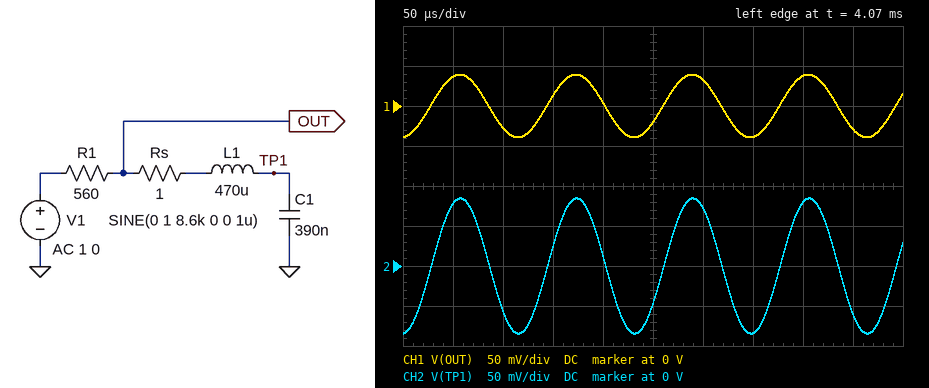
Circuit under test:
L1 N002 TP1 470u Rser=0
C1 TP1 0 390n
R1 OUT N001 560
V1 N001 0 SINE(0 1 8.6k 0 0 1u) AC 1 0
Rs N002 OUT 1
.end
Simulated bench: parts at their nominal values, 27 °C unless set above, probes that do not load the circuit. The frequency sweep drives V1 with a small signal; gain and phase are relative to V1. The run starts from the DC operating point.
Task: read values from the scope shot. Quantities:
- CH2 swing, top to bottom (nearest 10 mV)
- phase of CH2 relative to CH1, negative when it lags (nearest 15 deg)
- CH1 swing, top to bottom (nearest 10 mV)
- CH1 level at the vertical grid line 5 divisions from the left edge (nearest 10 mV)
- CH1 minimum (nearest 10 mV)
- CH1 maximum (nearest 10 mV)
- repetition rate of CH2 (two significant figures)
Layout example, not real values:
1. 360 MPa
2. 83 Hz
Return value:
1. 170 mV
2. 0 deg
3. 80 mV
4. -20 mV
5. -40 mV
6. 40 mV
7. 8.6 kHz
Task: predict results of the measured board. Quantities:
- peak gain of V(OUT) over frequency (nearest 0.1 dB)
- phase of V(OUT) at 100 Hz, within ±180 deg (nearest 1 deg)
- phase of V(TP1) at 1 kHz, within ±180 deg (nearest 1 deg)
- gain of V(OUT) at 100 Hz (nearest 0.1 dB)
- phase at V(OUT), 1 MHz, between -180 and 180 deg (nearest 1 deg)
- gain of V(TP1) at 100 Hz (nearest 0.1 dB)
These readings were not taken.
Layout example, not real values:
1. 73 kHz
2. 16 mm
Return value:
1. 0 dB
2. -8 deg
3. -54 deg
4. -0.1 dB
5. 11 deg
6. -0.1 dB
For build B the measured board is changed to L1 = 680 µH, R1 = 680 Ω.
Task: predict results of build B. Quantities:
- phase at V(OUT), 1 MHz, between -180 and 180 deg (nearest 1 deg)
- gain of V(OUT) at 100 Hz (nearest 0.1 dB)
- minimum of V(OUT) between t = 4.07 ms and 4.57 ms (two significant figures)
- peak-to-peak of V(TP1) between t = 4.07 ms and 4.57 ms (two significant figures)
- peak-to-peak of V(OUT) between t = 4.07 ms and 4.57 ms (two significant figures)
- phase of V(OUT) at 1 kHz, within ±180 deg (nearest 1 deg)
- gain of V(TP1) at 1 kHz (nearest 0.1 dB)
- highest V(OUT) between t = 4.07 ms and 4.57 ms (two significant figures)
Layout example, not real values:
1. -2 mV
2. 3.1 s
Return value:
1. 9 deg
2. -0.1 dB
3. -16 mV
4. 140 mV
5. 32 mV
6. -59 deg
7. -5.8 dB
8. 16 mV
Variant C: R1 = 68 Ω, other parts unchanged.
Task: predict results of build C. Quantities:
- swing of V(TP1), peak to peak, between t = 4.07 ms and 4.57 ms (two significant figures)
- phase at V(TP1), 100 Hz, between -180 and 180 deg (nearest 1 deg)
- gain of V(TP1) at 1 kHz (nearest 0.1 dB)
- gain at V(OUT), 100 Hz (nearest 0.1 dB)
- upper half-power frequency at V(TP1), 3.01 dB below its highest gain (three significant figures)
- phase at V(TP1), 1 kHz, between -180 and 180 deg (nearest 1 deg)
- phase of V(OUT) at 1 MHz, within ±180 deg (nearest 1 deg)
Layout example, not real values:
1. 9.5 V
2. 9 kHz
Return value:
1. 1.3 V
2. -1 deg
3. -0.1 dB
4. 0 dB
5. 7.63 kHz
6. -10 deg
7. 1 deg
